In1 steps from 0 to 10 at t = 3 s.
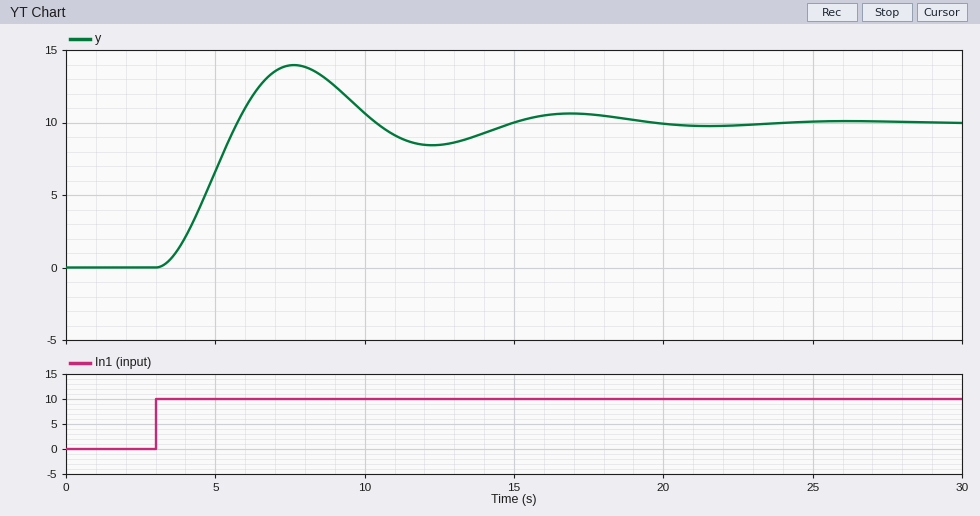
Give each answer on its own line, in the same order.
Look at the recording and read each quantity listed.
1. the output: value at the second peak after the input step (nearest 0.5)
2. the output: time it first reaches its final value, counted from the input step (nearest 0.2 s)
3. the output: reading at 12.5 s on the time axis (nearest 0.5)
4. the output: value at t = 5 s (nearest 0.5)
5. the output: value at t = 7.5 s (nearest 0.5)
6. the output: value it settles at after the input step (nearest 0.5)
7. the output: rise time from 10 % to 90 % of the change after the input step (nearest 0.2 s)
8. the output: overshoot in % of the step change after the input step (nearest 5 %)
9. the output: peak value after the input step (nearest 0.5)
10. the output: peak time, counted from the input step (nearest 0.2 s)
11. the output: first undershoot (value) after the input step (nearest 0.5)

10.5
2.8 s
8.5
6.5
14.0
10.0
1.8 s
40 %
14.0
4.6 s
8.5
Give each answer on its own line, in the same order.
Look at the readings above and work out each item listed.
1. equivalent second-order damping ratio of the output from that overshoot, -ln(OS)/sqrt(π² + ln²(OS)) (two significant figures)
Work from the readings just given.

0.28
